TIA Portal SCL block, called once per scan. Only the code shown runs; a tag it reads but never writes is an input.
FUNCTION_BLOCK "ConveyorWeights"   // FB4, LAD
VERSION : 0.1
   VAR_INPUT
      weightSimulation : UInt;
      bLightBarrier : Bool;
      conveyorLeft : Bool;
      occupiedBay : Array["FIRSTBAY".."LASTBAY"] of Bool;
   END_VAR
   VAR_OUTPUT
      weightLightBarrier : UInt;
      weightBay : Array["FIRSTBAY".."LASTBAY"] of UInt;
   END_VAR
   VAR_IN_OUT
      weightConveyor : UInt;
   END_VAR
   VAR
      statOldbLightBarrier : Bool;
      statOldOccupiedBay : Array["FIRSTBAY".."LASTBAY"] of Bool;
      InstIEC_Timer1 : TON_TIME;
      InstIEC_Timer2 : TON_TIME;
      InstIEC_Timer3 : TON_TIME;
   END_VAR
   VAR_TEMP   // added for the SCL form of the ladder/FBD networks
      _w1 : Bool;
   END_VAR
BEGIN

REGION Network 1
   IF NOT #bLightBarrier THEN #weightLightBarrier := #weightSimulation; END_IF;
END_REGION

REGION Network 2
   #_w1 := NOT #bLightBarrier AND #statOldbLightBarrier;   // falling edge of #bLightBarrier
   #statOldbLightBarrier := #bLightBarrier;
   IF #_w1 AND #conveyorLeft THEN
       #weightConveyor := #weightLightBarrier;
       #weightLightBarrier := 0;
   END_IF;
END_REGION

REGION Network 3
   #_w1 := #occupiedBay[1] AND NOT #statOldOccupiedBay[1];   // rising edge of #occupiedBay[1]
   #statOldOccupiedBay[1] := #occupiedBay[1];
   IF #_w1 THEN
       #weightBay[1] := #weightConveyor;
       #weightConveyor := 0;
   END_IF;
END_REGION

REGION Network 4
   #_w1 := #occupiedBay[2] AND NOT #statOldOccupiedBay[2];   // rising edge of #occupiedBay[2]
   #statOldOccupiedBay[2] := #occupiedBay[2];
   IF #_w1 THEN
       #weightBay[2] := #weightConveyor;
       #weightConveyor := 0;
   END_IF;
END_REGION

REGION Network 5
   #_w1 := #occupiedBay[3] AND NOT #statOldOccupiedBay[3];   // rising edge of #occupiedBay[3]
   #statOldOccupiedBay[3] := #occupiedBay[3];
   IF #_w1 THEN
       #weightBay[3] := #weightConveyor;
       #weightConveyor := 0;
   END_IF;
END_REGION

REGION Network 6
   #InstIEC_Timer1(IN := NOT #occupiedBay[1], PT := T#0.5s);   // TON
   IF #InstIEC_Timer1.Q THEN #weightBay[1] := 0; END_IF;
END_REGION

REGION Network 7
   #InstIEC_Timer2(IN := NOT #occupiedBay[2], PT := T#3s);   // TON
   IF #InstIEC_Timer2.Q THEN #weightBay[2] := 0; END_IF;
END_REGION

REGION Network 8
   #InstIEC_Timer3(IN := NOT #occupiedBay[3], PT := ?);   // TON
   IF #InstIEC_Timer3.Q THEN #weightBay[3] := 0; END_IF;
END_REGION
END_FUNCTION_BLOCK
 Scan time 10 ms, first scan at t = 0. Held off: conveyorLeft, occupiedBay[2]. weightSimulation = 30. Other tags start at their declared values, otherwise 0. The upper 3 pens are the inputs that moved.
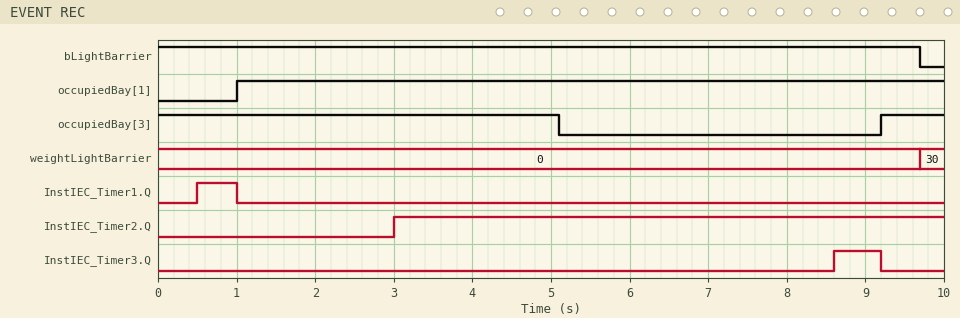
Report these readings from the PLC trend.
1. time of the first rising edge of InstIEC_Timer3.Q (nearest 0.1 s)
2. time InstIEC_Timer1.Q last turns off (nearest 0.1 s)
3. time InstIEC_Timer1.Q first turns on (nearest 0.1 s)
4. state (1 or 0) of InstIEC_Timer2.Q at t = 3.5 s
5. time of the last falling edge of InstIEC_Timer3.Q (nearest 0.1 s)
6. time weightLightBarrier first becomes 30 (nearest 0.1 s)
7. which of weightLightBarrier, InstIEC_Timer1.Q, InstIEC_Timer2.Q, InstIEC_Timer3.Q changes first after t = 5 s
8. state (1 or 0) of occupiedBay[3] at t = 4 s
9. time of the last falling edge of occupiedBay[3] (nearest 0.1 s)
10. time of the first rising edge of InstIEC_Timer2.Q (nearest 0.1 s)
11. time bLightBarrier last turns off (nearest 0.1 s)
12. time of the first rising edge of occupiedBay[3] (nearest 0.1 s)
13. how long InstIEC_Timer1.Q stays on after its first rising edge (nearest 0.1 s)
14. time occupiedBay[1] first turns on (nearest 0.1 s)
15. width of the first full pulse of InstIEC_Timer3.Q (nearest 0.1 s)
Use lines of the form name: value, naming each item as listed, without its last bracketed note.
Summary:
time of the first rising edge of InstIEC_Timer3.Q: 8.6 s
time InstIEC_Timer1.Q last turns off: 1.0 s
time InstIEC_Timer1.Q first turns on: 0.5 s
state (1 or 0) of InstIEC_Timer2.Q at t = 3.5 s: 1
time of the last falling edge of InstIEC_Timer3.Q: 9.2 s
time weightLightBarrier first becomes 30: 9.7 s
which of weightLightBarrier, InstIEC_Timer1.Q, InstIEC_Timer2.Q, InstIEC_Timer3.Q changes first after t = 5 s: InstIEC_Timer3.Q
state (1 or 0) of occupiedBay[3] at t = 4 s: 1
time of the last falling edge of occupiedBay[3]: 5.1 s
time of the first rising edge of InstIEC_Timer2.Q: 3.0 s
time bLightBarrier last turns off: 9.7 s
time of the first rising edge of occupiedBay[3]: 9.2 s
how long InstIEC_Timer1.Q stays on after its first rising edge: 0.5 s
time occupiedBay[1] first turns on: 1.0 s
width of the first full pulse of InstIEC_Timer3.Q: 0.6 s
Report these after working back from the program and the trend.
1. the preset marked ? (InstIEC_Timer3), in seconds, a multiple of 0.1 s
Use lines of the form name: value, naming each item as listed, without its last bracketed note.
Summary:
the preset marked ? (InstIEC_Timer3), in seconds, a multiple of 0.1 s: 3.5 s
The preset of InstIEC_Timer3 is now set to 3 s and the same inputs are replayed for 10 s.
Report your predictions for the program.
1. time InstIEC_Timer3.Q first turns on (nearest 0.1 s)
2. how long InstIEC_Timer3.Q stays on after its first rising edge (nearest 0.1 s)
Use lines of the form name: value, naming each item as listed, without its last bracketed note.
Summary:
time InstIEC_Timer3.Q first turns on: 8.1 s
how long InstIEC_Timer3.Q stays on after its first rising edge: 1.1 s
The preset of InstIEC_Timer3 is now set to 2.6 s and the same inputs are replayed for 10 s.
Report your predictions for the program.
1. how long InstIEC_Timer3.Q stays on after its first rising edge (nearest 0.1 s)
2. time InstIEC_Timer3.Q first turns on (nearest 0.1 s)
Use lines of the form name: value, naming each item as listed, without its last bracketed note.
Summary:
how long InstIEC_Timer3.Q stays on after its first rising edge: 1.5 s
time InstIEC_Timer3.Q first turns on: 7.7 s
